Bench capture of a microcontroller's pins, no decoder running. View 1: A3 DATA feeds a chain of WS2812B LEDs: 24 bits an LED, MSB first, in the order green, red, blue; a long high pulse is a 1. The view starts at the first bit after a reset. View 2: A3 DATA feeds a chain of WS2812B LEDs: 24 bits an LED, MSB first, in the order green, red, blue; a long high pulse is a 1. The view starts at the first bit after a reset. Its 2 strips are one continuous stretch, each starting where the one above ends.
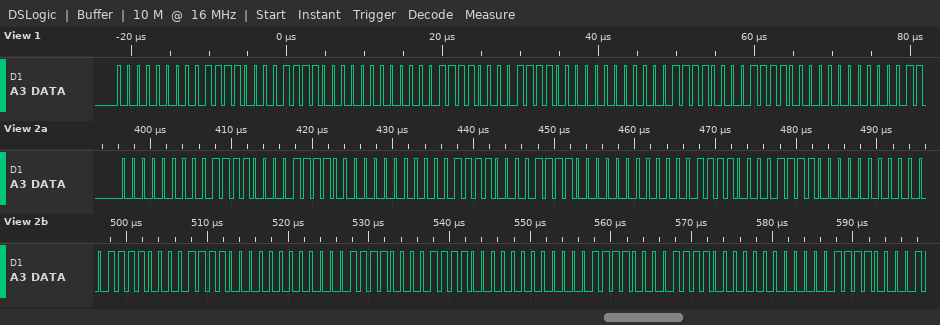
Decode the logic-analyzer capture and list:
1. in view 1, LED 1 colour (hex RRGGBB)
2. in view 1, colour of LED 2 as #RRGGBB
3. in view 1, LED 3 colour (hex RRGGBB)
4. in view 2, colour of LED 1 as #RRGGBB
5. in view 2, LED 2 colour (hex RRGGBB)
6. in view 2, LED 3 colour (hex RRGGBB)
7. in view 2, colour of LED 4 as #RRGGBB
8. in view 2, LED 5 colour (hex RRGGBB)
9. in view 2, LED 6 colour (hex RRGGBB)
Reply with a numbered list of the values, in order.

1. #780078
2. #780078
3. #780078
4. #780078
5. #780078
6. #780078
7. #780078
8. #780078
9. #780078
